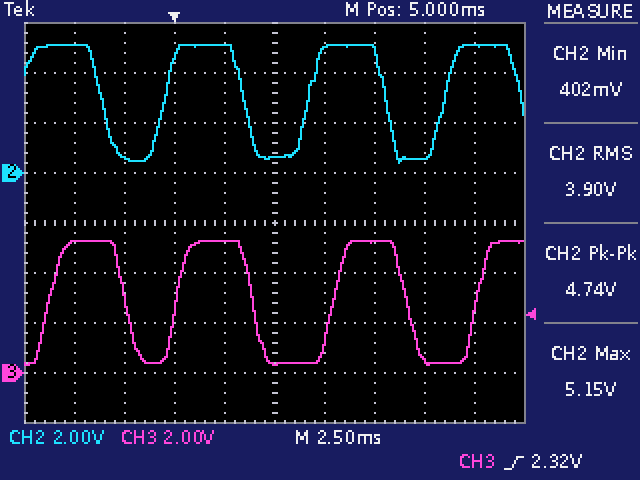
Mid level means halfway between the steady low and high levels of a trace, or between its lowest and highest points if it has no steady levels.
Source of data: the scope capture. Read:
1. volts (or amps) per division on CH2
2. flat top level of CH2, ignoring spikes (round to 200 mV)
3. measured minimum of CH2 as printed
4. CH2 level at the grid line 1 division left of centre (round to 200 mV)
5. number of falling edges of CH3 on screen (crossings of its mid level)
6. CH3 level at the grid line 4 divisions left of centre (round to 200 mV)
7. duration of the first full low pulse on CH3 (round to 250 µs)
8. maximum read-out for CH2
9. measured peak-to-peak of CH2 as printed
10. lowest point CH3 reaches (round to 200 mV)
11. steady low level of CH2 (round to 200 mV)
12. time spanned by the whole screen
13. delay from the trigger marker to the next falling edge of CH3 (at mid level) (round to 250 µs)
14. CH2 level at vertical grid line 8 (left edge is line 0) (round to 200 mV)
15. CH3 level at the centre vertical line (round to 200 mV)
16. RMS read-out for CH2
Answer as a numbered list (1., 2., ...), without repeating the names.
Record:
1. 2 V
2. 5.2 V
3. 402 mV
4. 5.2 V
5. 3
6. 5.2 V
7. 2.50 ms
8. 5.15 V
9. 4.74 V
10. 400 mV
11. 600 mV
12. 25 ms
13. 4.00 ms
14. 600 mV
15. 400 mV
16. 3.90 V
